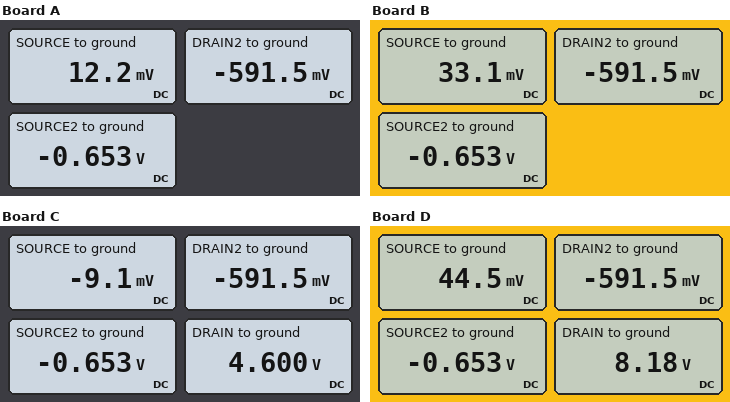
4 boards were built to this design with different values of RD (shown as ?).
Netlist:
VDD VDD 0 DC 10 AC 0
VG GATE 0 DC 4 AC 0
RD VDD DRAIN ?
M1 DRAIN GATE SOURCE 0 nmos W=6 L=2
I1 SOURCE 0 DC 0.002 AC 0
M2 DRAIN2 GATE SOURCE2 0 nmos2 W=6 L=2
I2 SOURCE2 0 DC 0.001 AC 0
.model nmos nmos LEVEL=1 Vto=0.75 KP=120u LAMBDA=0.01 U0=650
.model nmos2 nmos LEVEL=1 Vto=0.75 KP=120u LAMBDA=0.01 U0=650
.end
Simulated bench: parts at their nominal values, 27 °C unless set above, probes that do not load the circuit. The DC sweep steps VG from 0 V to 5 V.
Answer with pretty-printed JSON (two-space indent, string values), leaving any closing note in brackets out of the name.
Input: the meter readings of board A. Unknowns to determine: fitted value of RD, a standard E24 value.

{
  "fitted value of RD, a standard E24 value": "2 kΩ"
}
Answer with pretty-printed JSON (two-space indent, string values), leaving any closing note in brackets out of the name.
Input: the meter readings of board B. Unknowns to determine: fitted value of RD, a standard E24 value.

{
  "fitted value of RD, a standard E24 value": "1.3 kΩ"
}
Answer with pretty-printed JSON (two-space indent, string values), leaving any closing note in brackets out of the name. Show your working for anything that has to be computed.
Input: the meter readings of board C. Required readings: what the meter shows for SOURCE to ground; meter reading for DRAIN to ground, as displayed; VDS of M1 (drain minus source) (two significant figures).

{
  "what the meter shows for SOURCE to ground": "-9.1 mV",
  "meter reading for DRAIN to ground, as displayed": "4.600 V",
  "VDS of M1 (drain minus source)": "4.6 V - (-9.1 mV) = 4.6 V"
}
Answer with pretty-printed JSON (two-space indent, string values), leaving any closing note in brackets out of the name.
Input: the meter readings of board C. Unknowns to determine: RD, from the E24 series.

{
  "RD, from the E24 series": "2.7 kΩ"
}
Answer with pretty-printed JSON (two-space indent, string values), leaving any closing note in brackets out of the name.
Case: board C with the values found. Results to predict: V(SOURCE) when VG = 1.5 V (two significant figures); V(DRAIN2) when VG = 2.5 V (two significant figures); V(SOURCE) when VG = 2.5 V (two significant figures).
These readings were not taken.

{
  "V(SOURCE) when VG = 1.5 V": "-670 mV",
  "V(DRAIN2) when VG = 2.5 V": "-580 mV",
  "V(SOURCE) when VG = 2.5 V": "-650 mV"
}
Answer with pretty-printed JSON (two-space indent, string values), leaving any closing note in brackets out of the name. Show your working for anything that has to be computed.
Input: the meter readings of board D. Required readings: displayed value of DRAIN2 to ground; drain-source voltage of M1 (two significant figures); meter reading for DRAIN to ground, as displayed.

{
  "displayed value of DRAIN2 to ground": "-591.5 mV",
  "drain-source voltage of M1": "8.18 V - 44.5 mV = 8.1 V",
  "meter reading for DRAIN to ground, as displayed": "8.18 V"
}
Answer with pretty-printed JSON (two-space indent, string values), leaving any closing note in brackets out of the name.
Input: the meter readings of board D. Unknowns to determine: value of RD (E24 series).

{
  "value of RD": "910 Ω"
}
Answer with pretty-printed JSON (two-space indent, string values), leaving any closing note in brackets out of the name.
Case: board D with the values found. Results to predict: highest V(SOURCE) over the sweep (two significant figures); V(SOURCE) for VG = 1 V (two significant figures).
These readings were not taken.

{
  "highest V(SOURCE) over the sweep": "1.0 V",
  "V(SOURCE) for VG = 1 V": "-670 mV"
}
